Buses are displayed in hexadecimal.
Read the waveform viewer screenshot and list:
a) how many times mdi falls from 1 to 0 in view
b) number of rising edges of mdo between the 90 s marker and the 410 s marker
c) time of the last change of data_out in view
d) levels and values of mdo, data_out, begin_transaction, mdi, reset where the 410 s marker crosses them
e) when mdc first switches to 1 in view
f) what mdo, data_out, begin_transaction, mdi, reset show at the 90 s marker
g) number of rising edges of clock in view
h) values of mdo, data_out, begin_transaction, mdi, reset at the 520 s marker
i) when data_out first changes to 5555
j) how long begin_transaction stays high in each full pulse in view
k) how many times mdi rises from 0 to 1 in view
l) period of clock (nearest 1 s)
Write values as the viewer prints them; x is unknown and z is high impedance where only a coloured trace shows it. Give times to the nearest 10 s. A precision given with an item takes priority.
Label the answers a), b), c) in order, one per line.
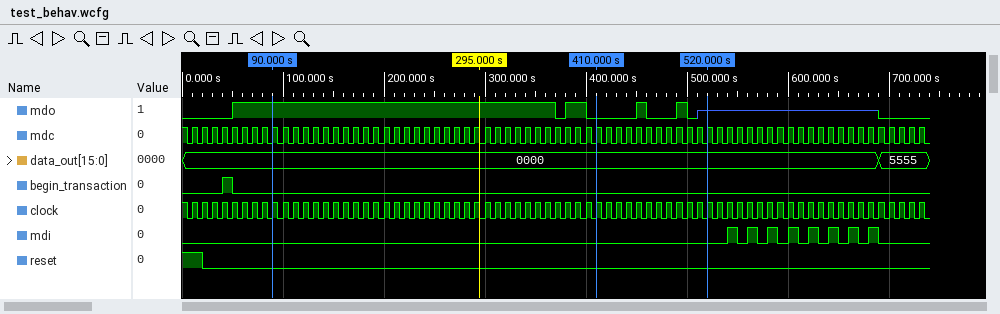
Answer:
a) 8
b) 1
c) 690 s
d) mdo=0, data_out=0000, begin_transaction=0, mdi=0, reset=0
e) 10 s
f) mdo=1, data_out=0000, begin_transaction=0, mdi=0, reset=0
g) 73
h) mdo=z, data_out=0000, begin_transaction=0, mdi=0, reset=0
i) 690 s
j) 10 s
k) 8
l) 10 s
